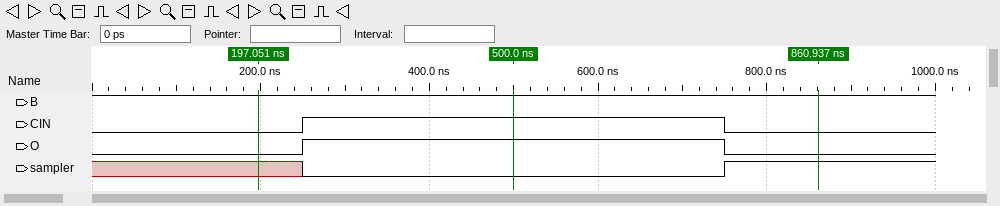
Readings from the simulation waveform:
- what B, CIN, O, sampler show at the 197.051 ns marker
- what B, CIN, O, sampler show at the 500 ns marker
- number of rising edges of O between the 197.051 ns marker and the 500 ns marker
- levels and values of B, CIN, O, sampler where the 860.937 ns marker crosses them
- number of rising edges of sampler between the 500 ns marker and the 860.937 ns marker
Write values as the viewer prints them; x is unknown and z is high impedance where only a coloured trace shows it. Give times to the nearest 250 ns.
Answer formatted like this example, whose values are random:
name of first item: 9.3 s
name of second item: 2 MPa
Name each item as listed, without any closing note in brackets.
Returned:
what B, CIN, O, sampler show at the 197.051 ns marker: B=1, CIN=0, O=0, sampler=x
what B, CIN, O, sampler show at the 500 ns marker: B=1, CIN=1, O=1, sampler=0
number of rising edges of O between the 197.051 ns marker and the 500 ns marker: 1
levels and values of B, CIN, O, sampler where the 860.937 ns marker crosses them: B=1, CIN=0, O=0, sampler=1
number of rising edges of sampler between the 500 ns marker and the 860.937 ns marker: 1
